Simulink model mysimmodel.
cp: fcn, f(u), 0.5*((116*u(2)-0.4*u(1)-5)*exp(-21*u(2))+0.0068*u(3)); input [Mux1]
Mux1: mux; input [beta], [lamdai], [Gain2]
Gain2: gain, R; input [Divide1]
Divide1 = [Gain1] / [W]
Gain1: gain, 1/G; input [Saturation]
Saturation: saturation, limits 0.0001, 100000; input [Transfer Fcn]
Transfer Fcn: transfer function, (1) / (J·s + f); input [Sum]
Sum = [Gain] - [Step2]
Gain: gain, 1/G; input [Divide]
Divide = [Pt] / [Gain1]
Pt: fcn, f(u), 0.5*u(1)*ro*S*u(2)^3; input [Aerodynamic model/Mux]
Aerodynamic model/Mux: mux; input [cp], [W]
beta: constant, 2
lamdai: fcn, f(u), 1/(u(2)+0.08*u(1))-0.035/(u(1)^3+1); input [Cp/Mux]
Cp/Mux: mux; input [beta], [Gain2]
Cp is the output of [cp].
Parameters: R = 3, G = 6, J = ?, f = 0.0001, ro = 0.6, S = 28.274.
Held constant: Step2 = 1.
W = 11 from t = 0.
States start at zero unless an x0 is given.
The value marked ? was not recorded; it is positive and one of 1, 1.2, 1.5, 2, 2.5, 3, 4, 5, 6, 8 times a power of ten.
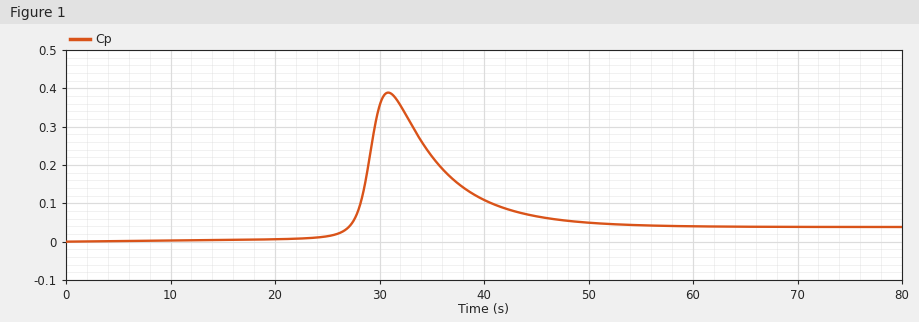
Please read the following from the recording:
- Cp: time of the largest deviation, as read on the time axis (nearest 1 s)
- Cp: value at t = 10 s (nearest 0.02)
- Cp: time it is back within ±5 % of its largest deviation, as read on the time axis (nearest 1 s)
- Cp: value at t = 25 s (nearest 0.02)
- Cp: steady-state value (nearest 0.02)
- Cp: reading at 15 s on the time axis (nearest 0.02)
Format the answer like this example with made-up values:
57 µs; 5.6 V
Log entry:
31 s; 0.00; 47 s; 0.02; 0.04; 0.00
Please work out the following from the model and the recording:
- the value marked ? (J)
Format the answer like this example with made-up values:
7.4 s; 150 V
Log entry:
0.4
